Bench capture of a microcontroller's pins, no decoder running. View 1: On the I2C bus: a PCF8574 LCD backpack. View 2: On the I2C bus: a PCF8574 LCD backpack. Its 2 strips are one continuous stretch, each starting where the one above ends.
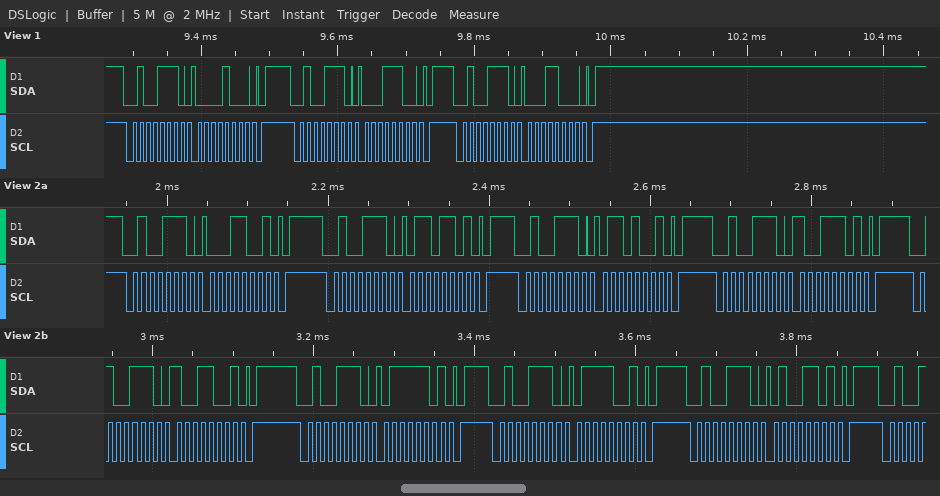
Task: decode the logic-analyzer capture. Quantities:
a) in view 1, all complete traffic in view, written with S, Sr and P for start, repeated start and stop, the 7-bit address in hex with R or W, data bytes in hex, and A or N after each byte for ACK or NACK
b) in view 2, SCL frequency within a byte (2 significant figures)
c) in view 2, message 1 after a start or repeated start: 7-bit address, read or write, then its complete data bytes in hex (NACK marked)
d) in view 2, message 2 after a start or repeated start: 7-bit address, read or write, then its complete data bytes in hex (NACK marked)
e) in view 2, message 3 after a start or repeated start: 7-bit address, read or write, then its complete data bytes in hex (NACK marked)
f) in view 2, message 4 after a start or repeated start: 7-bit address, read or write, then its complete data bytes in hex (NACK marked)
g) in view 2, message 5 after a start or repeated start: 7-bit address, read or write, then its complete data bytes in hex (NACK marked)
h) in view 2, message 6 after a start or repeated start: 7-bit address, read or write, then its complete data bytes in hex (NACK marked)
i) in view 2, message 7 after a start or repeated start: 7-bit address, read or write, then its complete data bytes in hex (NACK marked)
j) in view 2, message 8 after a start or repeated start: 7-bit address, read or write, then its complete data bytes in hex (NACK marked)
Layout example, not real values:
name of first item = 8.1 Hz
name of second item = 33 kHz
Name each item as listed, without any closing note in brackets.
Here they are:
in view 1, all complete traffic in view, written with S, Sr and P for start, repeated start and stop, the 7-bit address in hex with R or W, data bytes in hex, and A or N after each byte for ACK or NACK = S 27W A 08 A P S 27W A 1C A P S 27W A 18 A P
in view 2, SCL frequency within a byte = 100 kHz
in view 2, message 1 after a start or repeated start: 7-bit address, read or write, then its complete data bytes in hex = 0x27 write: 19
in view 2, message 2 after a start or repeated start: 7-bit address, read or write, then its complete data bytes in hex = 0x27 write: 6D
in view 2, message 3 after a start or repeated start: 7-bit address, read or write, then its complete data bytes in hex = 0x27 write: 69
in view 2, message 4 after a start or repeated start: 7-bit address, read or write, then its complete data bytes in hex = 0x27 write: 9D
in view 2, message 5 after a start or repeated start: 7-bit address, read or write, then its complete data bytes in hex = 0x27 write: 99
in view 2, message 6 after a start or repeated start: 7-bit address, read or write, then its complete data bytes in hex = 0x27 write: 7D
in view 2, message 7 after a start or repeated start: 7-bit address, read or write, then its complete data bytes in hex = 0x27 write: 79
in view 2, message 8 after a start or repeated start: 7-bit address, read or write, then its complete data bytes in hex = 0x27 write: 4D
